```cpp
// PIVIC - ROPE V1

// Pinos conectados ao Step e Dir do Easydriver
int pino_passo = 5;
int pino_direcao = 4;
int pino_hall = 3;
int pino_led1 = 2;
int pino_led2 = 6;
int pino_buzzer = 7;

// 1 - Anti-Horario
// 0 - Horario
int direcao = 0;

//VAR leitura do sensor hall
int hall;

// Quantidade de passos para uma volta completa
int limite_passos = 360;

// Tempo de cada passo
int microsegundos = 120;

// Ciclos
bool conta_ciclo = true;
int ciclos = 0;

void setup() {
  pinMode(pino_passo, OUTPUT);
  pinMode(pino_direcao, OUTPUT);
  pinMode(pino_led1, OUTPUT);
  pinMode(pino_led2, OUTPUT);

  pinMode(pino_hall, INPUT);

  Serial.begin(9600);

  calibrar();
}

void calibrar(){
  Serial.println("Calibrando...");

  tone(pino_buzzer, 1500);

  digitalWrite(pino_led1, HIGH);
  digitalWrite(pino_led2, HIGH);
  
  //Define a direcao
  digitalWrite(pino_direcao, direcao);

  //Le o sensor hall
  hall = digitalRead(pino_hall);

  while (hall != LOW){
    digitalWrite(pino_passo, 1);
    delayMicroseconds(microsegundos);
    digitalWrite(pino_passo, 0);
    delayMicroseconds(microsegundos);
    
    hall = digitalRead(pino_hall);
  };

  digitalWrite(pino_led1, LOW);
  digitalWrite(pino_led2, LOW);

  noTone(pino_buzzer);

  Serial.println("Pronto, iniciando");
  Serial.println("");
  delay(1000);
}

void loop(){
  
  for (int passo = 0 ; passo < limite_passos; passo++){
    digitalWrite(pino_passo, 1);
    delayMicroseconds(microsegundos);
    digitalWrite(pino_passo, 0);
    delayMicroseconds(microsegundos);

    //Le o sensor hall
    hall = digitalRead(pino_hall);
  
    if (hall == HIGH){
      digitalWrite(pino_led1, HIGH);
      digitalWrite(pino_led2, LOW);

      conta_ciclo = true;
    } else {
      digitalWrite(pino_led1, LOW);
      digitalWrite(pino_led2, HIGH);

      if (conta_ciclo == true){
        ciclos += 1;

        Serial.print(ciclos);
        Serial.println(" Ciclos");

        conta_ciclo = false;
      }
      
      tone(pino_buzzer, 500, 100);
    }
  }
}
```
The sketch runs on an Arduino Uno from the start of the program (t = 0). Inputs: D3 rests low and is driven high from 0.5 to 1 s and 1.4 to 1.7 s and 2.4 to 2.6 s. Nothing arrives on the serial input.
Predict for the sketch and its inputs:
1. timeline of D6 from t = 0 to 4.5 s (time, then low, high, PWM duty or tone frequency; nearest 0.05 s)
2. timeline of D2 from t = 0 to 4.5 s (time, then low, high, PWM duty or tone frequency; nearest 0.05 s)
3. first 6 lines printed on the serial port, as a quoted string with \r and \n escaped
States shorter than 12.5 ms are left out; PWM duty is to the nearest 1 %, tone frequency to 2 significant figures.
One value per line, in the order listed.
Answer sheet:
0 s low; 1 s high; 1.4 s low; 1.7 s high; 2.4 s low; 2.6 s high
0 s low; 1.4 s high; 1.7 s low; 2.4 s high; 2.6 s low
"Calibrando...\r\nPronto, iniciando\r\n\r\n1 Ciclos\r\n2 Ciclos\r\n3 Ciclos\r\n"
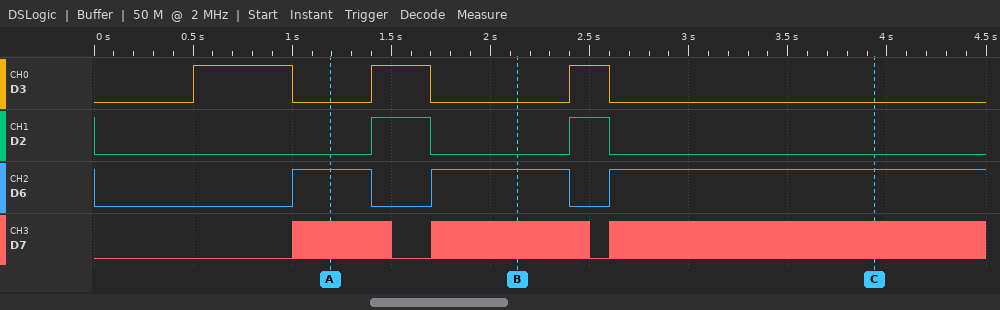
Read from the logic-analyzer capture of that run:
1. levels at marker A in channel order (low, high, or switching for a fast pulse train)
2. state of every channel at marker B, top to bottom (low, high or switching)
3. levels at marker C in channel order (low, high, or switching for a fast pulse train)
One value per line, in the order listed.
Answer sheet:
D3 low, D2 low, D6 high, D7 switching
D3 low, D2 low, D6 high, D7 switching
D3 low, D2 low, D6 high, D7 switching
